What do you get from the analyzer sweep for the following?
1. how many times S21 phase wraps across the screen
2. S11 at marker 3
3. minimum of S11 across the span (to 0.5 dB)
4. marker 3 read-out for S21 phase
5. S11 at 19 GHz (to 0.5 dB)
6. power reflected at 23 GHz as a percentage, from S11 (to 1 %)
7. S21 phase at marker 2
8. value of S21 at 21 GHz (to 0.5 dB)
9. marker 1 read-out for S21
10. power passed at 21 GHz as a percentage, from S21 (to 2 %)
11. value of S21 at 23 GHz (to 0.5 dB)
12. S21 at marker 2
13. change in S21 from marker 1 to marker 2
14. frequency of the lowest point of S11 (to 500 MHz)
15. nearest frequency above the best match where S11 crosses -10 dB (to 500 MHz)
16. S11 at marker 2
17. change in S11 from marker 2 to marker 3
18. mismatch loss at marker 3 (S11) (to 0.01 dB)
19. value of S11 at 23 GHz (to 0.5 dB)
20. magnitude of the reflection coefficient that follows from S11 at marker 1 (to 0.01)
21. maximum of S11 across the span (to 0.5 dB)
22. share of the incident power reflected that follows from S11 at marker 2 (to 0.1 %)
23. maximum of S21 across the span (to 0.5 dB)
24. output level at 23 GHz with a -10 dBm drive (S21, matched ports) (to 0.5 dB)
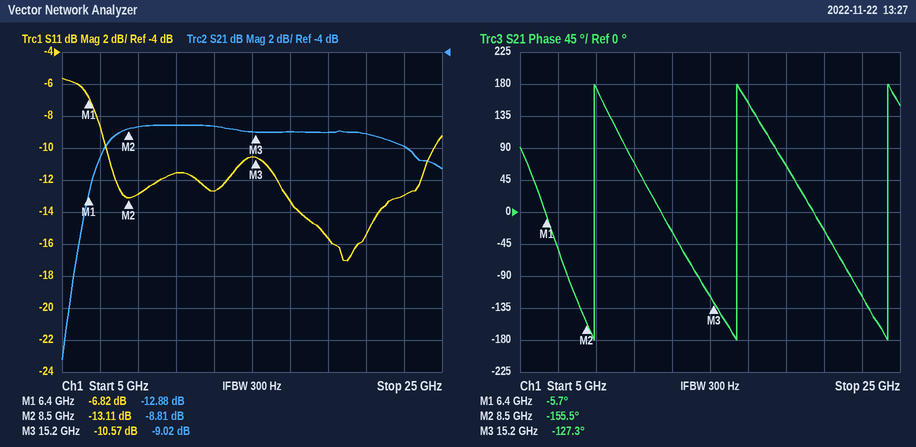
3
-10.57 dB
-17.0 dB
-127.3°
-15.5 dB
5 %
-155.5°
-9.0 dB
-12.88 dB
12 %
-10.0 dB
-8.81 dB
4.07 dB
20.0 GHz
24.5 GHz
-13.11 dB
2.54 dB
0.40 dB
-13.0 dB
0.46
-5.5 dB
4.9 %
-8.5 dB
-20.0 dBm
